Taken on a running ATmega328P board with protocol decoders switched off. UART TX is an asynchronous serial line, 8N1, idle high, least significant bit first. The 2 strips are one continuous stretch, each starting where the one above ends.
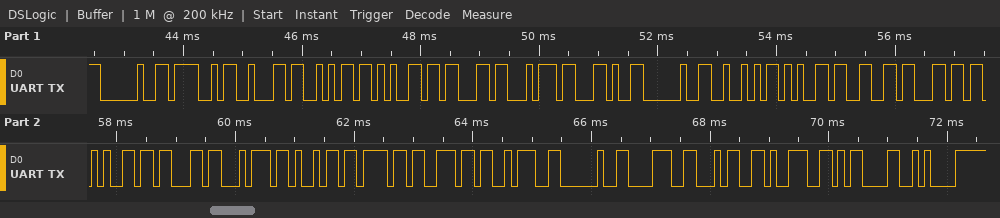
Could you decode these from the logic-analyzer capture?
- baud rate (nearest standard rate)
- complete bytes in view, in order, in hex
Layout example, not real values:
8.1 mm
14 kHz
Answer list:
9600 baud
20 4F 62 6A 65 63 74 2C 20 52 65 66 6C 65 63 74 69 6F 6E 3A 20 38 34 39 0D 0A
